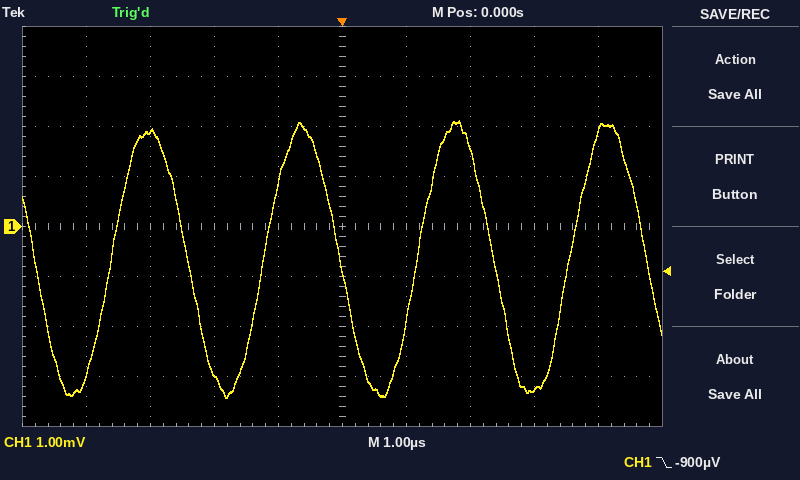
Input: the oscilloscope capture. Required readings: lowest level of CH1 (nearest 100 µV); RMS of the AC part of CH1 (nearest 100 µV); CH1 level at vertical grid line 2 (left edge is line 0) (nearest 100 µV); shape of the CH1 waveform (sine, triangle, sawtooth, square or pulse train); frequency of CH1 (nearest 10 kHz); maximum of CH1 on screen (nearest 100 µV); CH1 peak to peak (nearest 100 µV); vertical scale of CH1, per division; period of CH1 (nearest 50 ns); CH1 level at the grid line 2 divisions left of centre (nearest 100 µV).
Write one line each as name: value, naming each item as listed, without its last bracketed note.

lowest level of CH1: -3.4 mV
RMS of the AC part of CH1: 1.9 mV
CH1 level at vertical grid line 2 (left edge is line 0): 1.9 mV
shape of the CH1 waveform: sine
frequency of CH1: 420 kHz
maximum of CH1 on screen: 2.1 mV
CH1 peak to peak: 5.5 mV
vertical scale of CH1, per division: 1 mV
period of CH1: 2.40 µs
CH1 level at the grid line 2 divisions left of centre: -2.9 mV
